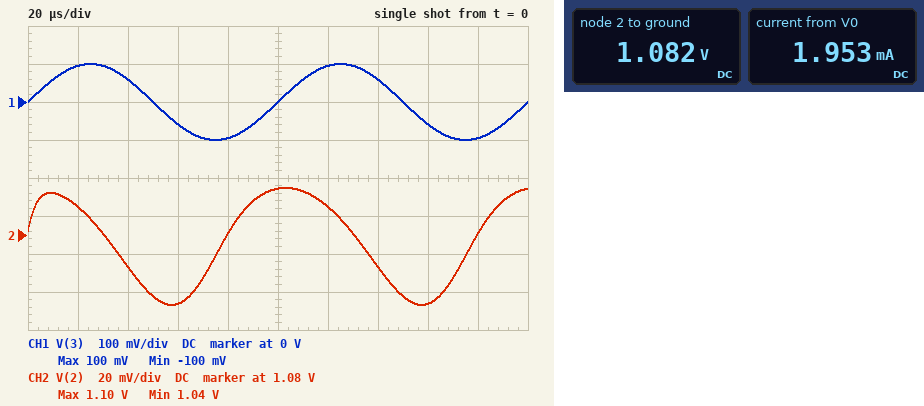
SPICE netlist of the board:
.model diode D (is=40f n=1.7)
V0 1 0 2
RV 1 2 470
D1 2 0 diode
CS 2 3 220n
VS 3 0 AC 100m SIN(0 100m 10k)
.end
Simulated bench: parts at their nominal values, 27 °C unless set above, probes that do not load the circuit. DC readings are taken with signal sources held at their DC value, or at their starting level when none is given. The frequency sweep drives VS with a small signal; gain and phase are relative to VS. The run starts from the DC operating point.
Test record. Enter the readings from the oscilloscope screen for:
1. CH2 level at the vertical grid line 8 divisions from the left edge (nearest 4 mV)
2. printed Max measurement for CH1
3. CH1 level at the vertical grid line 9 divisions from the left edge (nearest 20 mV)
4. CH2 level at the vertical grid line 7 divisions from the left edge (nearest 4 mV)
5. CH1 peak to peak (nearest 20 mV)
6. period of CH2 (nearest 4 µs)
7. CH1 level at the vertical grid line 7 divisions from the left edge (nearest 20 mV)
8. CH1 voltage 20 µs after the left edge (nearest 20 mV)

1.044 V
100 mV
-100 mV
1.064 V
200 mV
100 µs
60 mV
100 mV
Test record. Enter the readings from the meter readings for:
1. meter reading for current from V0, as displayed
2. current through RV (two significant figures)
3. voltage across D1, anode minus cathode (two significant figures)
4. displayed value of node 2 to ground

1.953 mA
2.0 mA
1.1 V
1.082 V
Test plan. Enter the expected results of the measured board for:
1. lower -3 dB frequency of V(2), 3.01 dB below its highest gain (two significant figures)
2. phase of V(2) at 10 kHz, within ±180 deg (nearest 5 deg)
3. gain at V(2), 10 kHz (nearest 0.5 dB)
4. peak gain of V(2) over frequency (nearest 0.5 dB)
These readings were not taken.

34 kHz
75 deg
-11.0 dB
0 dB
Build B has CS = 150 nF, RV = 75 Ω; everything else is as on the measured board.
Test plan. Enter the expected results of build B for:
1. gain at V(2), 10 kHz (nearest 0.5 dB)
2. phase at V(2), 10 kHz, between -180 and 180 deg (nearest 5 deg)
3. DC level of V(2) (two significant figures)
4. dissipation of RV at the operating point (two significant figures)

-29.0 dB
90 deg
1.2 V
9.4 mW
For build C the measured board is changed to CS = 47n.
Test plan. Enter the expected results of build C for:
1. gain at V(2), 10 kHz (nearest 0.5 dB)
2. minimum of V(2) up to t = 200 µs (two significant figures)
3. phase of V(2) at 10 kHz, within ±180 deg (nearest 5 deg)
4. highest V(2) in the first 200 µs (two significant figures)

-24.0 dB
1.1 V
85 deg
1.1 V
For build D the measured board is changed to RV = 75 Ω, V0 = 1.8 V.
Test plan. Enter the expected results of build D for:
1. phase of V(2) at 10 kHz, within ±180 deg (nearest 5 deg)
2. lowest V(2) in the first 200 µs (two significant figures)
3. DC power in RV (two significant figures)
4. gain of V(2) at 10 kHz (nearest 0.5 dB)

85 deg
1.1 V
5.7 mW
-23.5 dB
